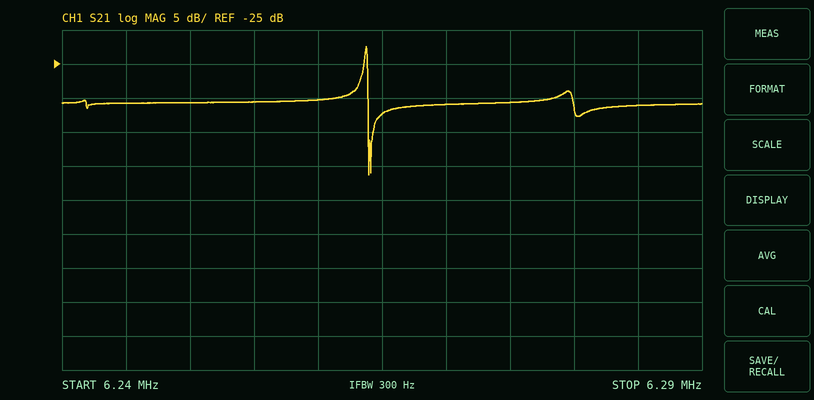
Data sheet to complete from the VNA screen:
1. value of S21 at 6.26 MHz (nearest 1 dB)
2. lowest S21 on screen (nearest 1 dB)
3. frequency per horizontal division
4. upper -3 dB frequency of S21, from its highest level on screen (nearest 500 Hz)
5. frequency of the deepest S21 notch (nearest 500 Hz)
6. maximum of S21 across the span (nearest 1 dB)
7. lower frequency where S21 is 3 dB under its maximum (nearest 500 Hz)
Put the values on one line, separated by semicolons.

-30 dB; -41 dB; 5 kHz; 6.2640 MHz; 6.2640 MHz; -22 dB; 6.2635 MHz
